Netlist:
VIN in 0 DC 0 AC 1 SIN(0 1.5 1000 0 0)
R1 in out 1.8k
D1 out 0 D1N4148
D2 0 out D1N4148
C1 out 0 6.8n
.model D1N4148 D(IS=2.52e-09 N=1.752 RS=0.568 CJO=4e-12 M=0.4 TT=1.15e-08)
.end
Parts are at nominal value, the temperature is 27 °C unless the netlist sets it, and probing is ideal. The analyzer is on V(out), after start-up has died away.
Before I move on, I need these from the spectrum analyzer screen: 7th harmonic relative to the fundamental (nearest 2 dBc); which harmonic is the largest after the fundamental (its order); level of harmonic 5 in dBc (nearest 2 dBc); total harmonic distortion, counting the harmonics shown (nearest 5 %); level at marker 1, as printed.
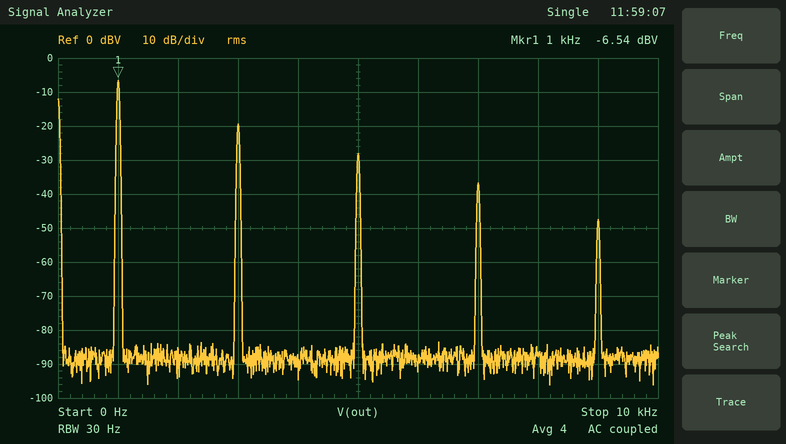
-30 dBc
3
-22 dBc
25 %
-6.54 dBV
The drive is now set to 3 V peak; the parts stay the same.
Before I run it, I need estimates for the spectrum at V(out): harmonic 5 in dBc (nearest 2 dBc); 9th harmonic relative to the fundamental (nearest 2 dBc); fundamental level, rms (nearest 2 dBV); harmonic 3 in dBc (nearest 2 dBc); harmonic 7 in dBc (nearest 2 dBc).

-18 dBc
-26 dBc
-6 dBV
-12 dBc
-22 dBc
